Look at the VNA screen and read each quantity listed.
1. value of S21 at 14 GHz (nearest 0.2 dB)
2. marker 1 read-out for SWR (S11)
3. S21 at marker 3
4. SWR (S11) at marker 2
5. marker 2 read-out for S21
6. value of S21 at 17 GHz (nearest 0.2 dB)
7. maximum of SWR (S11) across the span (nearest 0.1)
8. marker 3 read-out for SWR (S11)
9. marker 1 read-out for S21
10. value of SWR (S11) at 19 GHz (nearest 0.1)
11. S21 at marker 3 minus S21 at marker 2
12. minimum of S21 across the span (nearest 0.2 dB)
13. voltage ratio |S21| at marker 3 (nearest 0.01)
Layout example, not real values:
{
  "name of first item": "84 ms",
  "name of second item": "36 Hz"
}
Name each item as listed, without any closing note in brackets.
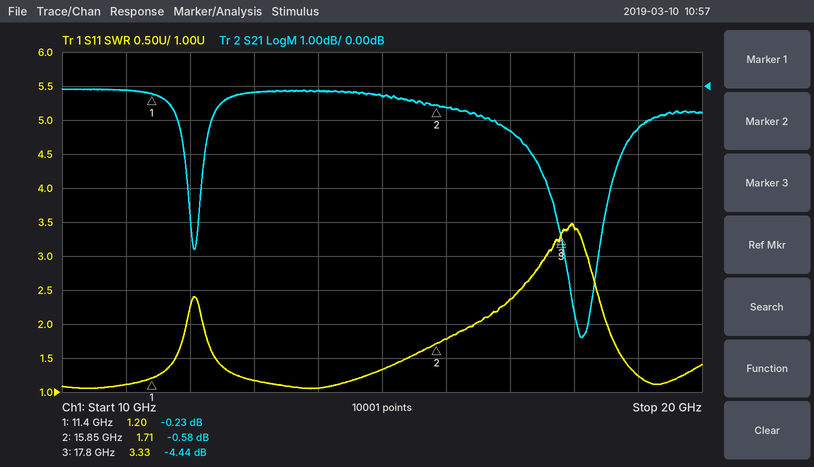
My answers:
{
  "value of S21 at 14 GHz": "-0.2 dB",
  "marker 1 read-out for SWR": "1.20",
  "S21 at marker 3": "-4.44 dB",
  "SWR (S11) at marker 2": "1.71",
  "marker 2 read-out for S21": "-0.58 dB",
  "value of S21 at 17 GHz": "-1.4 dB",
  "maximum of SWR (S11) across the span": "3.5",
  "marker 3 read-out for SWR": "3.33",
  "marker 1 read-out for S21": "-0.23 dB",
  "value of SWR (S11) at 19 GHz": "1.2",
  "S21 at marker 3 minus S21 at marker 2": "-3.86 dB",
  "minimum of S21 across the span": "-7.4 dB",
  "voltage ratio |S21| at marker 3": "0.60"
}
